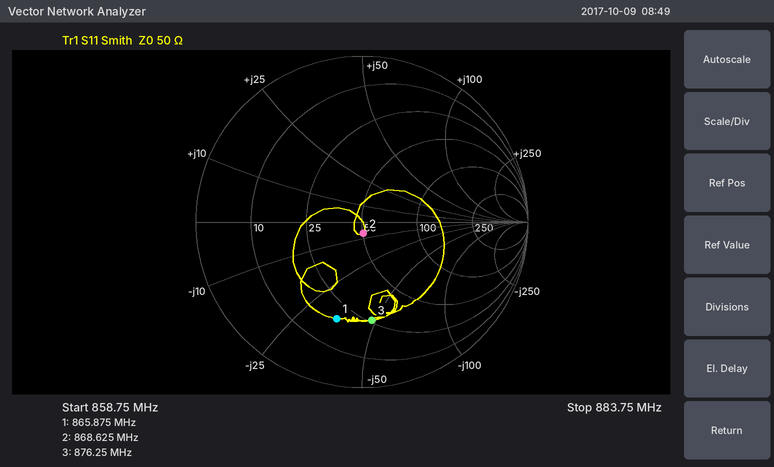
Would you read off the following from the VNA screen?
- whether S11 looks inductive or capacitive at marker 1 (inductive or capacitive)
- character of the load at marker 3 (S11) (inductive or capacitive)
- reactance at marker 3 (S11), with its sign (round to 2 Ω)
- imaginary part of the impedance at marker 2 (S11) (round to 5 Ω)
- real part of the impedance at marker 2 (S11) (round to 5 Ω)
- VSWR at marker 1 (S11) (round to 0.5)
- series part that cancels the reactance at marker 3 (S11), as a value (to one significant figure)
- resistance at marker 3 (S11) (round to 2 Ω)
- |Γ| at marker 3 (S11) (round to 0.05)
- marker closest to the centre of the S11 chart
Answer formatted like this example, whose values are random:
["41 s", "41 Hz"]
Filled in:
["capacitive", "capacitive", "-48 Ω", "-5 Ω", "50 Ω", "4.0", "9 nH", "26 Ω", "0.60", "marker 2"]
